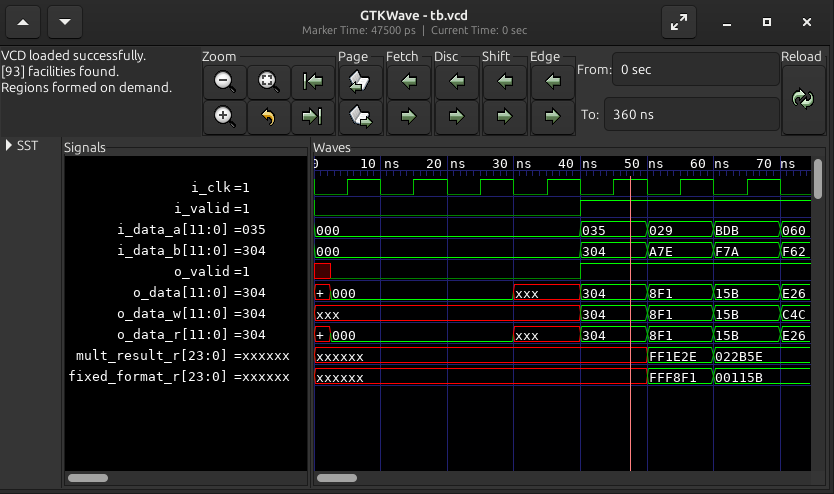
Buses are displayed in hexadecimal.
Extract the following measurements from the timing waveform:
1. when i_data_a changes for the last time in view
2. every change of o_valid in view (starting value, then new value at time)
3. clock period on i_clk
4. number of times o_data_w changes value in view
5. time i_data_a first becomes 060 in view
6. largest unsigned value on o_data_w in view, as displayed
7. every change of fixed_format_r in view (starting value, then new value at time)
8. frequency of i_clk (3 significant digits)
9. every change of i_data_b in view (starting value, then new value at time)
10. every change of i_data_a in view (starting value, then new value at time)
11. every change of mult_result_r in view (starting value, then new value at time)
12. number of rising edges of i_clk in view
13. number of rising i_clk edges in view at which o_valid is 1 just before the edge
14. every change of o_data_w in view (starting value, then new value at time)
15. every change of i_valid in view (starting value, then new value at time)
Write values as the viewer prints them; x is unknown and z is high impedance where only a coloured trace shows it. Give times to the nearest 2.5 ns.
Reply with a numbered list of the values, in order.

1. 70 ns
2. x, 0 at 2.5 ns, 1 at 40 ns
3. 10 ns
4. 4
5. 70 ns
6. C4C
7. xxxxxx, FFF8F1 at 50 ns, 00115B at 60 ns
8. 100 MHz
9. 000, 304 at 40 ns, A7E at 50 ns, F7A at 60 ns, F62 at 70 ns
10. 000, 035 at 40 ns, 029 at 50 ns, BDB at 60 ns, 060 at 70 ns
11. xxxxxx, FF1E2E at 50 ns, 022B5E at 60 ns
12. 7
13. 3
14. xxx, 304 at 40 ns, 8F1 at 50 ns, 15B at 60 ns, C4C at 70 ns
15. 0, 1 at 40 ns
